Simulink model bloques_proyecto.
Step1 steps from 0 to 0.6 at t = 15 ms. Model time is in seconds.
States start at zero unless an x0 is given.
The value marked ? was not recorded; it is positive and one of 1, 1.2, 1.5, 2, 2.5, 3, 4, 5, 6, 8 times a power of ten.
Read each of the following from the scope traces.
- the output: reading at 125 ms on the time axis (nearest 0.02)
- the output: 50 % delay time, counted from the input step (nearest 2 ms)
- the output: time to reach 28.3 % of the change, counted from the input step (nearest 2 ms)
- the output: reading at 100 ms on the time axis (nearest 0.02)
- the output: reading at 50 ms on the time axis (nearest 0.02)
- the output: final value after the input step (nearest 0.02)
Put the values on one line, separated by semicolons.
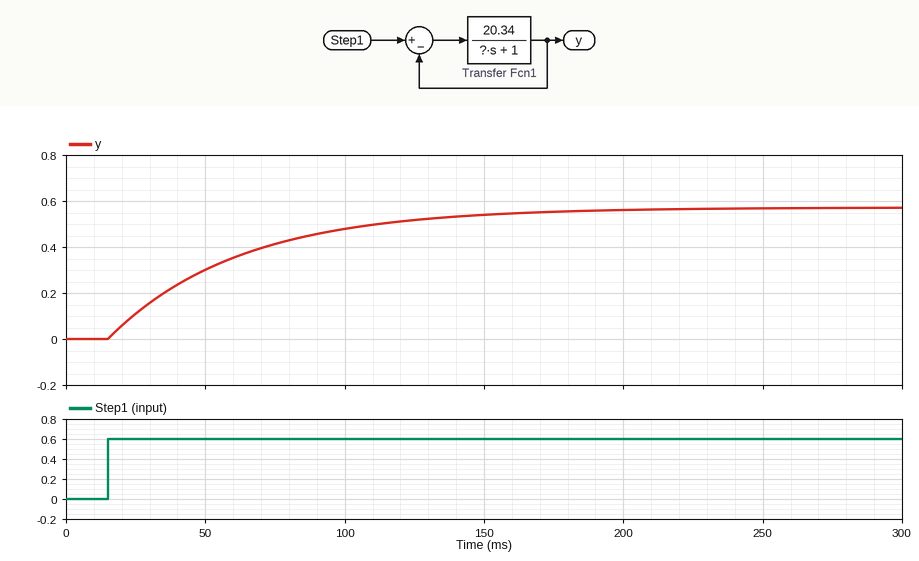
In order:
0.52; 32 ms; 16 ms; 0.48; 0.30; 0.58
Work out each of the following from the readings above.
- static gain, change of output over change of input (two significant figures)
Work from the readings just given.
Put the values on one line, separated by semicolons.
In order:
0.97
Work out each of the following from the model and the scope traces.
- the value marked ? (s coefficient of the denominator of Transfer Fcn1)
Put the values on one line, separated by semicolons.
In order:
1
